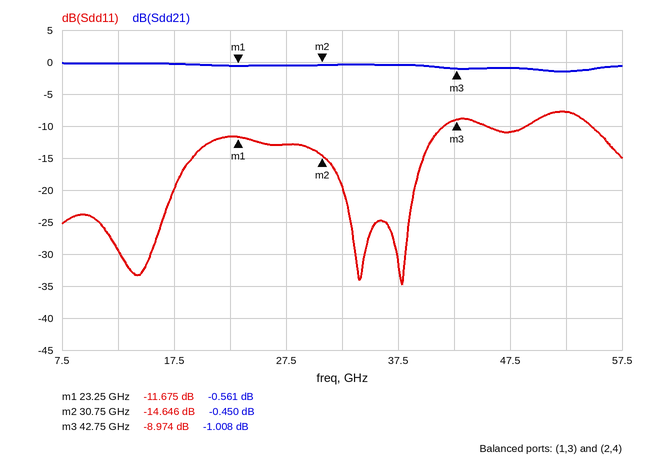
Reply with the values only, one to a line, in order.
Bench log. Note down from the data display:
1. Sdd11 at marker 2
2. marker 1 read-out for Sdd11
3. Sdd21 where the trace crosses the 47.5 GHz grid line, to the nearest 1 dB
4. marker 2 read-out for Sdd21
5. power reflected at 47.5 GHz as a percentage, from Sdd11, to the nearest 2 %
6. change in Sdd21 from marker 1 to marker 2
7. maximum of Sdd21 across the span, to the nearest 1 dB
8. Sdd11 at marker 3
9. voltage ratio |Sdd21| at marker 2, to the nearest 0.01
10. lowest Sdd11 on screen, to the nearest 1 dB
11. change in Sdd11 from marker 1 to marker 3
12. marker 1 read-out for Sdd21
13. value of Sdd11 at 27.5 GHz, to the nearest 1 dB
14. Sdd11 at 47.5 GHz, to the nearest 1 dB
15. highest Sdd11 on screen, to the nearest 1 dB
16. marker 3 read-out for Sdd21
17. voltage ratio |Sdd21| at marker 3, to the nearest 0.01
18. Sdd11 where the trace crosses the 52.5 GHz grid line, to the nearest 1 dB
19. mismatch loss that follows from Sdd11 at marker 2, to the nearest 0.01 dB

-14.646 dB
-11.675 dB
-1 dB
-0.450 dB
8 %
0.111 dB
0 dB
-8.974 dB
0.95
-35 dB
2.701 dB
-0.561 dB
-13 dB
-11 dB
-8 dB
-1.008 dB
0.89
-8 dB
0.15 dB
